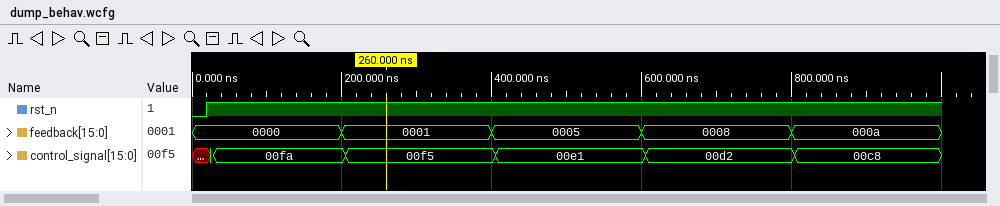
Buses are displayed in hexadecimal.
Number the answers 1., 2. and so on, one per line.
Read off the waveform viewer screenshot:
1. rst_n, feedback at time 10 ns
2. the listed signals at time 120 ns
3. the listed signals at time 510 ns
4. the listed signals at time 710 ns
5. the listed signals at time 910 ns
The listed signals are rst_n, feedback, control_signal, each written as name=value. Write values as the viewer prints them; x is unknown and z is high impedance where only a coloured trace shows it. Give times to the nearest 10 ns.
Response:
1. rst_n=0, feedback=0000
2. rst_n=1, feedback=0000, control_signal=00fa
3. rst_n=1, feedback=0005, control_signal=00e1
4. rst_n=1, feedback=0008, control_signal=00d2
5. rst_n=1, feedback=000a, control_signal=00c8
